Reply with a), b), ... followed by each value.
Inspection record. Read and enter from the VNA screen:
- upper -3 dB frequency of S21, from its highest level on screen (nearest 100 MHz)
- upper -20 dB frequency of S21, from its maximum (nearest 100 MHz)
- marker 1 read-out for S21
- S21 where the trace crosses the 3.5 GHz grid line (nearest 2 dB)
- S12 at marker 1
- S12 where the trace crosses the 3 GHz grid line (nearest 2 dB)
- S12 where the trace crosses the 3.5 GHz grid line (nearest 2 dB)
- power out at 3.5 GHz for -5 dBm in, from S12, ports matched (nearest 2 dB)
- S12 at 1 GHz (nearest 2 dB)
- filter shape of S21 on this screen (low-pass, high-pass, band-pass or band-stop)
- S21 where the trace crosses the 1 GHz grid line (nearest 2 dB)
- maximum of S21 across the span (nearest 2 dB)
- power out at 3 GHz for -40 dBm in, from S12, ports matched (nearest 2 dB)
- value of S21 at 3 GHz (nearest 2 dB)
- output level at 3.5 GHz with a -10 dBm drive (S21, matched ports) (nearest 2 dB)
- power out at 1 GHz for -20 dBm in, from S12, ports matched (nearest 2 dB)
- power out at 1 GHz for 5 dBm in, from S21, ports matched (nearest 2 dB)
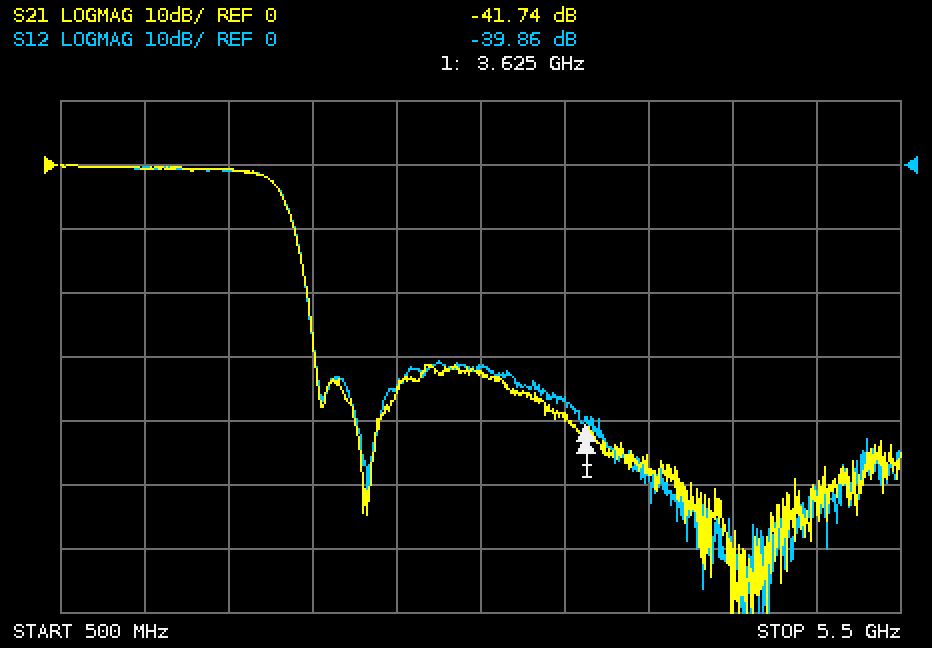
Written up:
a) 1.8 GHz
b) 2.0 GHz
c) -41.74 dB
d) -40 dB
e) -39.86 dB
f) -32 dB
g) -36 dB
h) -42 dBm
i) 0 dB
j) low-pass
k) 0 dB
l) 0 dB
m) -72 dBm
n) -32 dB
o) -50 dBm
p) -20 dBm
q) 4 dBm
